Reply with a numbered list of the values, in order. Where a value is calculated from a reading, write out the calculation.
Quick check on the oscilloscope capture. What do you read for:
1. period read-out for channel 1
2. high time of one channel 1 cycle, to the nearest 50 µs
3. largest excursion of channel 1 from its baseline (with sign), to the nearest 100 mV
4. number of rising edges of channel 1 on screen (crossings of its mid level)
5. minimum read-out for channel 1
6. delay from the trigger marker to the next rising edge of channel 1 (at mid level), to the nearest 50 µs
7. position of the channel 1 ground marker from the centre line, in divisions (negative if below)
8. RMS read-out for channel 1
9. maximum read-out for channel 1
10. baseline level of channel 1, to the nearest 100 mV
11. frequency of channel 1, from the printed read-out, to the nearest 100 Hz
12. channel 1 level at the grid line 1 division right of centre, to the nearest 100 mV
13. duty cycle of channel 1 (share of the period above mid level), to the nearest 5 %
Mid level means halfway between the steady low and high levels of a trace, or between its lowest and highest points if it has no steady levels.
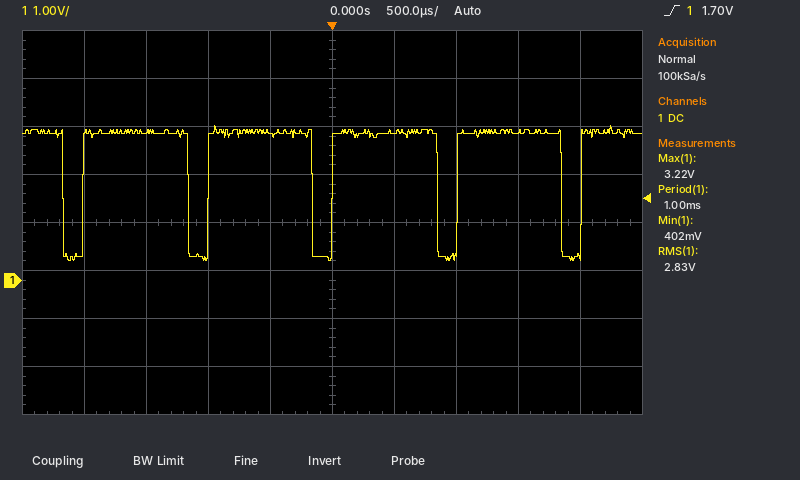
1. 1.00 ms
2. 850 µs
3. -2.7 V
4. 5
5. 402 mV
6. 1.00 ms
7. -1.2 div
8. 2.83 V
9. 3.22 V
10. 3.1 V
11. 1 / 1.00 ms ≈ 1.0 kHz
12. 3.1 V
13. 85 %
